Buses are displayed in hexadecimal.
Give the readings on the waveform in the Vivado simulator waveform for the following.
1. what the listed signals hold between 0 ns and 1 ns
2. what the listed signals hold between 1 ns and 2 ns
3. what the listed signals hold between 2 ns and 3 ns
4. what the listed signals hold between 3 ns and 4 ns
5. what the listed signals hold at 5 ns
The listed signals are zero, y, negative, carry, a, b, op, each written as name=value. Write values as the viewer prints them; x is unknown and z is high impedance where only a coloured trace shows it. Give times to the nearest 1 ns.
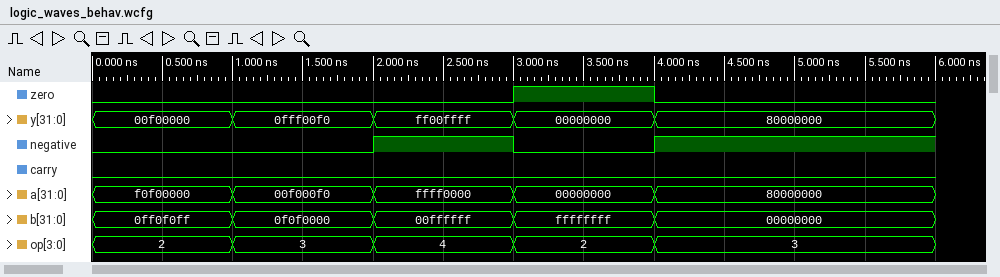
zero=0, y=00f00000, negative=0, carry=0, a=f0f00000, b=0ff0f0ff, op=2
zero=0, y=0fff00f0, negative=0, carry=0, a=00f000f0, b=0f0f0000, op=3
zero=0, y=ff00ffff, negative=1, carry=0, a=ffff0000, b=00ffffff, op=4
zero=1, y=00000000, negative=0, carry=0, a=00000000, b=ffffffff, op=2
zero=0, y=80000000, negative=1, carry=0, a=80000000, b=00000000, op=3
